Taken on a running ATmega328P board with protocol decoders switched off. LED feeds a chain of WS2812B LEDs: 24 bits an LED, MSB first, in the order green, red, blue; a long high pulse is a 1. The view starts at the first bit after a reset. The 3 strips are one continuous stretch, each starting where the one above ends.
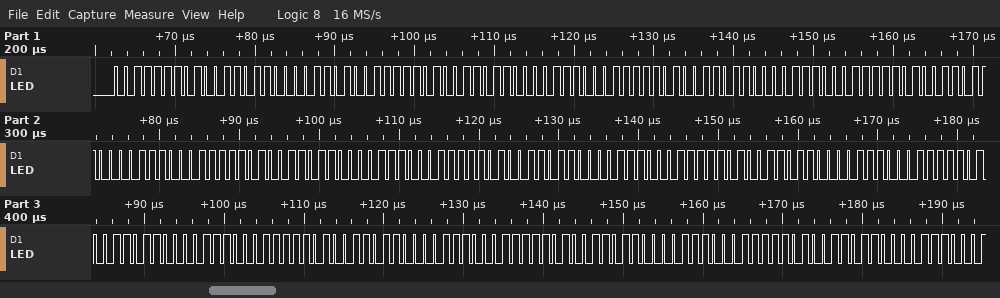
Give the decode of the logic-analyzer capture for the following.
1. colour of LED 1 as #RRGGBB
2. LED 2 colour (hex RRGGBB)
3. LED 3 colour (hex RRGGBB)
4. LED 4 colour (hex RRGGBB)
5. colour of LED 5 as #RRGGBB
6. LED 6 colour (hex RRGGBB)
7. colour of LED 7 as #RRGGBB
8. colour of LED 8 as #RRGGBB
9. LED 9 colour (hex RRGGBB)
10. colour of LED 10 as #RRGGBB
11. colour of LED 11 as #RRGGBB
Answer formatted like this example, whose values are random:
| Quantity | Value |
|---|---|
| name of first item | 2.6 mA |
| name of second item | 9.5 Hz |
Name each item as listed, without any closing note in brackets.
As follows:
| Quantity | Value |
|---|---|
| colour of LED 1 as #RRGGBB | #9B3E0D |
| LED 2 colour | #9B3E0E |
| LED 3 colour | #9B3E0E |
| LED 4 colour | #9B3E0E |
| colour of LED 5 as #RRGGBB | #9B3E0E |
| LED 6 colour | #9B3E0E |
| colour of LED 7 as #RRGGBB | #9B3E0E |
| colour of LED 8 as #RRGGBB | #9B3E0E |
| LED 9 colour | #9B3E0E |
| colour of LED 10 as #RRGGBB | #9B3E0E |
| colour of LED 11 as #RRGGBB | #9B3E0E |
